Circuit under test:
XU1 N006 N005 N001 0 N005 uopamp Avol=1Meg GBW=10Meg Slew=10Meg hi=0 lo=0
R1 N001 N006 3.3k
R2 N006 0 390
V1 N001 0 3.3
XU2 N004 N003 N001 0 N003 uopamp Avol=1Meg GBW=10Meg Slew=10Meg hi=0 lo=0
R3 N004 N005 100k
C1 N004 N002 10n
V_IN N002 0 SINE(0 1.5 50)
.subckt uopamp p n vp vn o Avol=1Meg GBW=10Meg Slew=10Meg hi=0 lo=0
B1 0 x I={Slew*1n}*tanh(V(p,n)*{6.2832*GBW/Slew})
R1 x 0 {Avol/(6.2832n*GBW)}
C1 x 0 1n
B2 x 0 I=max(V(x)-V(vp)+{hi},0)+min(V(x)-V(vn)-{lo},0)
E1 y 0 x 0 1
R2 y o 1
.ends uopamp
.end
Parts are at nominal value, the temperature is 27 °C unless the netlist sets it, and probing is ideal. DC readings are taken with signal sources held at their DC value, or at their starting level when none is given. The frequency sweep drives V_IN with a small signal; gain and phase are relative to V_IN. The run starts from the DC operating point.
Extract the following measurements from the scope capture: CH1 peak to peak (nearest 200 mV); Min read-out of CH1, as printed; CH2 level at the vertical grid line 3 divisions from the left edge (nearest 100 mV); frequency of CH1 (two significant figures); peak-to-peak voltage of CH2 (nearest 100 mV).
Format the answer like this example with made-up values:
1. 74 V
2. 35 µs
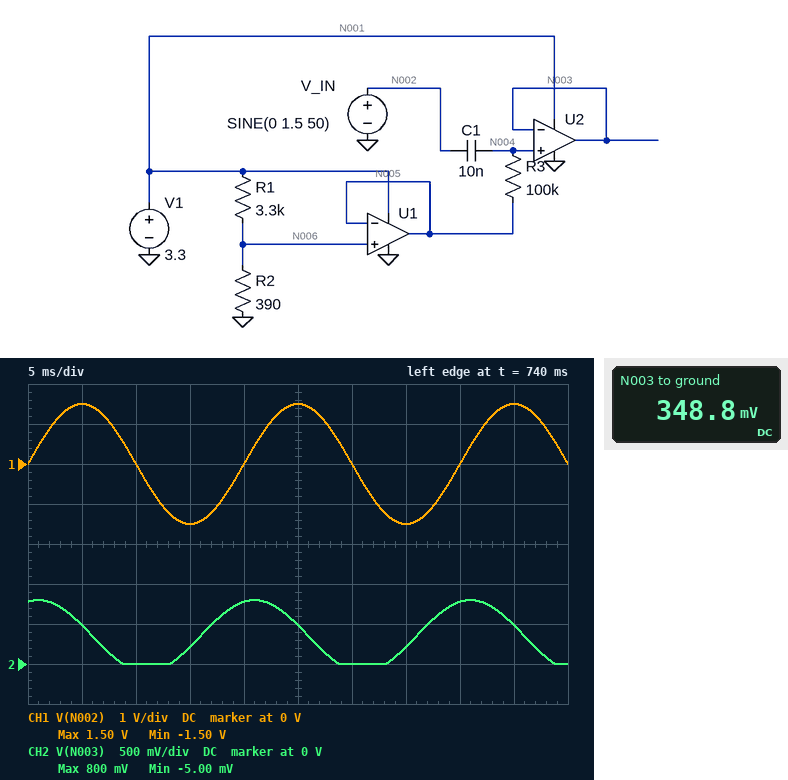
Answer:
1. 3.0 V
2. -1.50 V
3. 200 mV
4. 50 Hz
5. 800 mV
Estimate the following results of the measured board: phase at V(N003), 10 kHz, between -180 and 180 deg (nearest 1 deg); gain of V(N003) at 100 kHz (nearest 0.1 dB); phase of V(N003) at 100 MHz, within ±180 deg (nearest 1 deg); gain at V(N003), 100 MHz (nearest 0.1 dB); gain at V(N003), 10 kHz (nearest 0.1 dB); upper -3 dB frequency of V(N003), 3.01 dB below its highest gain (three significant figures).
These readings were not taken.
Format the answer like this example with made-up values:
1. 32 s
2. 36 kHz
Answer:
1. 1 deg
2. 0 dB
3. -84 deg
4. -20.0 dB
5. 0 dB
6. 10.0 MHz
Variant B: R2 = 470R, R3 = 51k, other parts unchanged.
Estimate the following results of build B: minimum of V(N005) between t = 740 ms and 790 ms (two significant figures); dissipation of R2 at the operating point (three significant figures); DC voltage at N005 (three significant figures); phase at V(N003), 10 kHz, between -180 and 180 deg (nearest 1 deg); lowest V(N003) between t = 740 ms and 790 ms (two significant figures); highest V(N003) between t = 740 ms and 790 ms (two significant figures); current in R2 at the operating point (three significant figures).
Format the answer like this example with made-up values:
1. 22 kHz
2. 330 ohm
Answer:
1. 410 mV
2. 360 µW
3. 411 mV
4. 2 deg
5. 170 mV
6. 650 mV
7. 875 µA
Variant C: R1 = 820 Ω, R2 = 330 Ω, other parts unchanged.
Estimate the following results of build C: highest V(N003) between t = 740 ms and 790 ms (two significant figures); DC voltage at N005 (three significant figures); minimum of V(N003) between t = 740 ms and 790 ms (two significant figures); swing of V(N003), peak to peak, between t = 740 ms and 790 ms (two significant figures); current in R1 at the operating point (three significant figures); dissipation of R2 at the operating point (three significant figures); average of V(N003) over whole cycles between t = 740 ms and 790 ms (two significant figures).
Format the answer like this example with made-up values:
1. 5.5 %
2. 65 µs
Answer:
1. 1.4 V
2. 947 mV
3. 500 mV
4. 900 mV
5. 2.87 mA
6. 2.72 mW
7. 950 mV
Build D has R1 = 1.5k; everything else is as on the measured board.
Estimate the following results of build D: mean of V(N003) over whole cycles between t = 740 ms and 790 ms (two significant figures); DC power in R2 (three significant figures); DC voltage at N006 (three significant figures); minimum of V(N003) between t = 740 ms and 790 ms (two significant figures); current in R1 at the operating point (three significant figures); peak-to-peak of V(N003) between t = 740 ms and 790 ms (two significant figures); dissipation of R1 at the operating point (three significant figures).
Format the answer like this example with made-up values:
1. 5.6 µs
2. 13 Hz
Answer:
1. 680 mV
2. 1.19 mW
3. 681 mV
4. 230 mV
5. 1.75 mA
6. 900 mV
7. 4.57 mW
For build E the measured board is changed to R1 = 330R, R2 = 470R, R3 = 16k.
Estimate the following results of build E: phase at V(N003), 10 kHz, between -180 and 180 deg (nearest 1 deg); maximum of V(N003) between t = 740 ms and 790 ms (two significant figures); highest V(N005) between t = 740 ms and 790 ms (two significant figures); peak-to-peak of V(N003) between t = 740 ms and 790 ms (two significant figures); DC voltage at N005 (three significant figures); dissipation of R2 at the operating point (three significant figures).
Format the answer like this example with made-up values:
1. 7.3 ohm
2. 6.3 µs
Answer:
1. 6 deg
2. 2.0 V
3. 1.9 V
4. 150 mV
5. 1.94 V
6. 8.00 mW
